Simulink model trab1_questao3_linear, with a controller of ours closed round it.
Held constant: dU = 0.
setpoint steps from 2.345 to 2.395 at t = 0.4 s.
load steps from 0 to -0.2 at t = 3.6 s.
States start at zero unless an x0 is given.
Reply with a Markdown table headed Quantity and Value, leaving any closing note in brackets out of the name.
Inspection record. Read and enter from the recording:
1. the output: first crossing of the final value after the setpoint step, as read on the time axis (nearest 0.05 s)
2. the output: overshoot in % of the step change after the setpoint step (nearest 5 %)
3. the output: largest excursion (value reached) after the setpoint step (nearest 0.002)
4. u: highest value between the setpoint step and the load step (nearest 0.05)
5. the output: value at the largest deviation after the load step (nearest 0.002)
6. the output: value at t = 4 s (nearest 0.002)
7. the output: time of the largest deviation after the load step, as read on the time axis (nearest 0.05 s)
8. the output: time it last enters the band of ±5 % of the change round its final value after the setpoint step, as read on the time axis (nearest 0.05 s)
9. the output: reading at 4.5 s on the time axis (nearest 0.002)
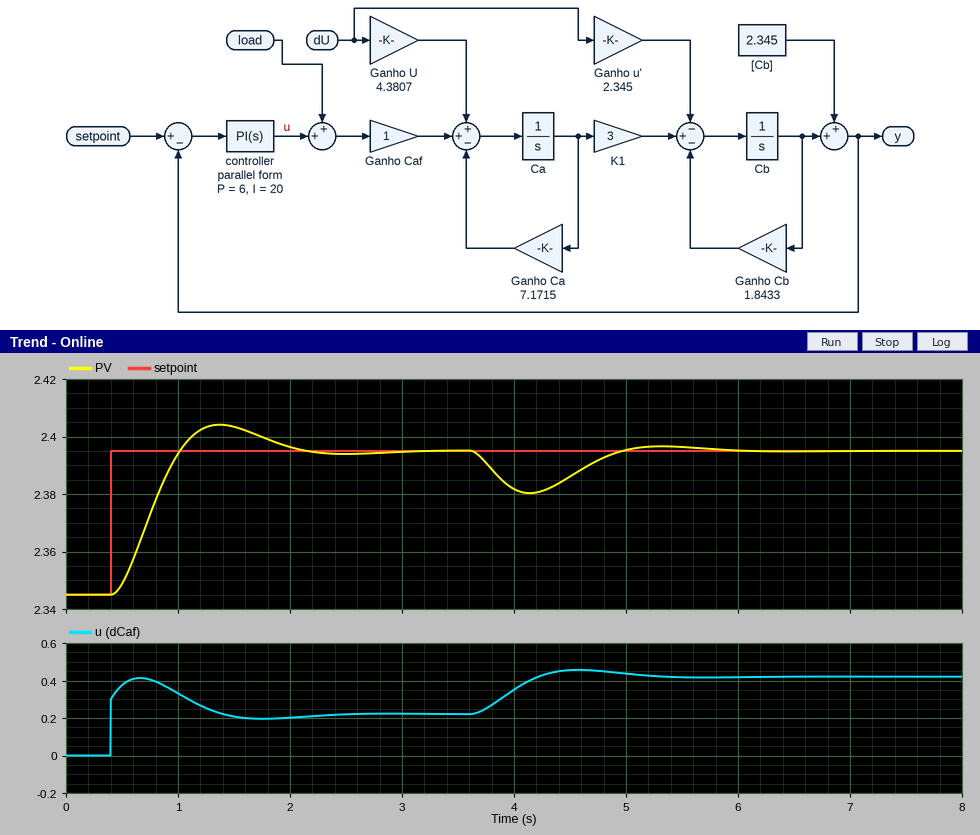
| Quantity | Value |
|---|---|
| the output: first crossing of the final value after the setpoint step, as read on the time axis | 1.00 s |
| the output: overshoot in % of the step change after the setpoint step | 20 % |
| the output: largest excursion (value reached) after the setpoint step | 2.404 |
| u: highest value between the setpoint step and the load step | 0.40 |
| the output: value at the largest deviation after the load step | 2.380 |
| the output: value at t = 4 s | 2.382 |
| the output: time of the largest deviation after the load step, as read on the time axis | 4.15 s |
| the output: time it last enters the band of ±5 % of the change round its final value after the setpoint step, as read on the time axis | 1.90 s |
| the output: reading at 4.5 s on the time axis | 2.386 |
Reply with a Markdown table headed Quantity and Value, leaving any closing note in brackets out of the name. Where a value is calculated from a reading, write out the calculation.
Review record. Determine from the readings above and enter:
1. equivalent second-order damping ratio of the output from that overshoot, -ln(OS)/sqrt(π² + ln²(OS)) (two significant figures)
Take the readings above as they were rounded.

| Quantity | Value |
|---|---|
| equivalent second-order damping ratio of the output from that overshoot, -ln(OS)/sqrt(π² + ln²(OS)) | ln(0.2) = -1.609; 1.609 / sqrt(9.870 + 2.590) = 0.46 |
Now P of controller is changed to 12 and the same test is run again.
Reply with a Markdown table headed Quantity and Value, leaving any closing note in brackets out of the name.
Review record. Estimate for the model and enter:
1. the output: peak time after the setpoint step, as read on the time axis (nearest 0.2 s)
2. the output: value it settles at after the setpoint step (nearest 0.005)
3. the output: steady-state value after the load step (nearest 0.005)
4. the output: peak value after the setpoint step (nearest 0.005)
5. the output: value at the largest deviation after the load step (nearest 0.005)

| Quantity | Value |
|---|---|
| the output: peak time after the setpoint step, as read on the time axis | 1.0 s |
| the output: value it settles at after the setpoint step | 2.395 |
| the output: steady-state value after the load step | 2.395 |
| the output: peak value after the setpoint step | 2.400 |
| the output: value at the largest deviation after the load step | 2.385 |
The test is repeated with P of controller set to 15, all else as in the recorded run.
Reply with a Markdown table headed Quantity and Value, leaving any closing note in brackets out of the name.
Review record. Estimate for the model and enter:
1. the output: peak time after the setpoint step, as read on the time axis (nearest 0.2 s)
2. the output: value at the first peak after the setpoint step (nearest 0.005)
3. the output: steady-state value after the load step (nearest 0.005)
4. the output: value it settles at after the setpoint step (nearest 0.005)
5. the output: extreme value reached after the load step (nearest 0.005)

| Quantity | Value |
|---|---|
| the output: peak time after the setpoint step, as read on the time axis | 1.0 s |
| the output: value at the first peak after the setpoint step | 2.400 |
| the output: steady-state value after the load step | 2.395 |
| the output: value it settles at after the setpoint step | 2.395 |
| the output: extreme value reached after the load step | 2.385 |
